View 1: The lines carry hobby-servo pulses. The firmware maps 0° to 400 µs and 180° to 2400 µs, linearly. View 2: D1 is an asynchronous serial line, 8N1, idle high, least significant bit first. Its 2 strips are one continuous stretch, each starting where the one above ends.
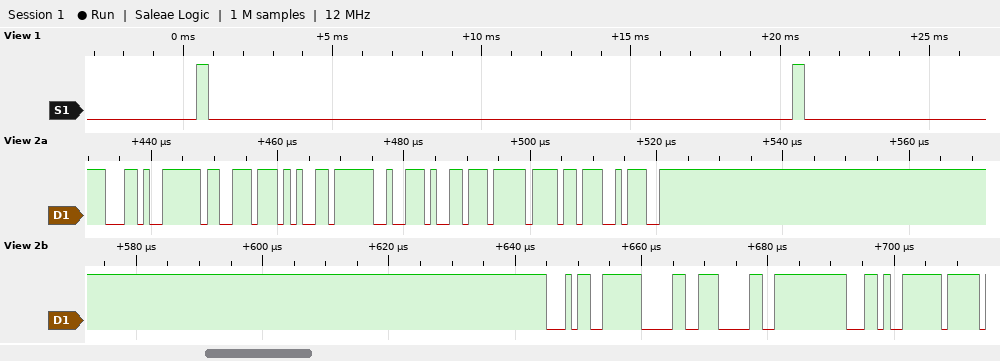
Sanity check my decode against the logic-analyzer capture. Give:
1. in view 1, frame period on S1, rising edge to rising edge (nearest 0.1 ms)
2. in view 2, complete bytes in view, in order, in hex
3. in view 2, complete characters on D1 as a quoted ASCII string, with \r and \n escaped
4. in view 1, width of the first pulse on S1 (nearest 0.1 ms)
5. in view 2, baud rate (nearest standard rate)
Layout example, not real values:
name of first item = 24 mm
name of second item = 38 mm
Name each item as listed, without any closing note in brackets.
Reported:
in view 1, frame period on S1, rising edge to rising edge = 20.0 ms
in view 2, complete bytes in view, in order, in hex = 2C 73 65 72 76 6F 3A 34 30 30 2C
in view 2, complete characters on D1 as a quoted ASCII string, with \r and \n escaped = ",servo:400,"
in view 1, width of the first pulse on S1 = 0.4 ms
in view 2, baud rate = 1000000 baud
